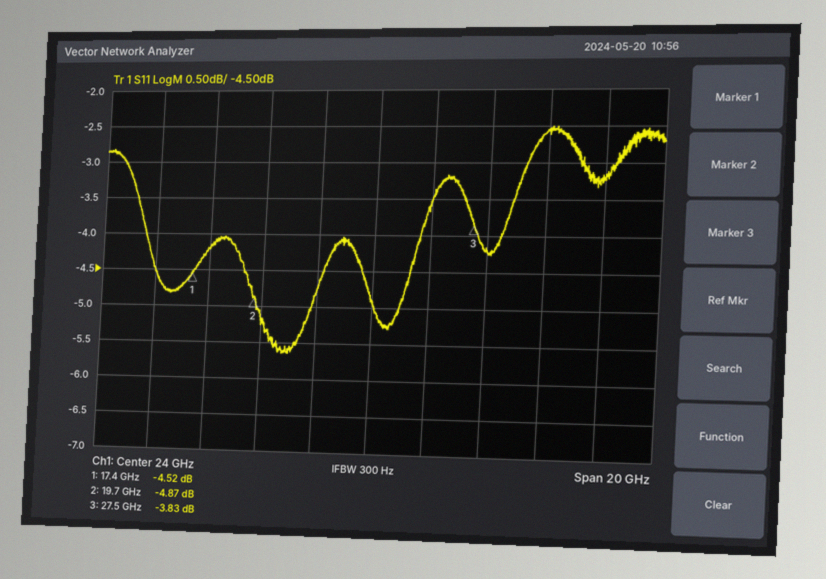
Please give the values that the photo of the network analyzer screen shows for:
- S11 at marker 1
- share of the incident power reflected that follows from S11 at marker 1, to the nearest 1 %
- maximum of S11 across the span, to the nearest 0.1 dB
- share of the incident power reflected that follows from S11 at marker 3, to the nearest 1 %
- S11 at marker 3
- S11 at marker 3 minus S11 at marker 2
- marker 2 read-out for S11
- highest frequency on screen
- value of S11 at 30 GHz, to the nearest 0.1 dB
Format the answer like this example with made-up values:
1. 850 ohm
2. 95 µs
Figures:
1. -4.52 dB
2. 35 %
3. -2.5 dB
4. 41 %
5. -3.83 dB
6. 1.04 dB
7. -4.87 dB
8. 34 GHz
9. -2.6 dB
